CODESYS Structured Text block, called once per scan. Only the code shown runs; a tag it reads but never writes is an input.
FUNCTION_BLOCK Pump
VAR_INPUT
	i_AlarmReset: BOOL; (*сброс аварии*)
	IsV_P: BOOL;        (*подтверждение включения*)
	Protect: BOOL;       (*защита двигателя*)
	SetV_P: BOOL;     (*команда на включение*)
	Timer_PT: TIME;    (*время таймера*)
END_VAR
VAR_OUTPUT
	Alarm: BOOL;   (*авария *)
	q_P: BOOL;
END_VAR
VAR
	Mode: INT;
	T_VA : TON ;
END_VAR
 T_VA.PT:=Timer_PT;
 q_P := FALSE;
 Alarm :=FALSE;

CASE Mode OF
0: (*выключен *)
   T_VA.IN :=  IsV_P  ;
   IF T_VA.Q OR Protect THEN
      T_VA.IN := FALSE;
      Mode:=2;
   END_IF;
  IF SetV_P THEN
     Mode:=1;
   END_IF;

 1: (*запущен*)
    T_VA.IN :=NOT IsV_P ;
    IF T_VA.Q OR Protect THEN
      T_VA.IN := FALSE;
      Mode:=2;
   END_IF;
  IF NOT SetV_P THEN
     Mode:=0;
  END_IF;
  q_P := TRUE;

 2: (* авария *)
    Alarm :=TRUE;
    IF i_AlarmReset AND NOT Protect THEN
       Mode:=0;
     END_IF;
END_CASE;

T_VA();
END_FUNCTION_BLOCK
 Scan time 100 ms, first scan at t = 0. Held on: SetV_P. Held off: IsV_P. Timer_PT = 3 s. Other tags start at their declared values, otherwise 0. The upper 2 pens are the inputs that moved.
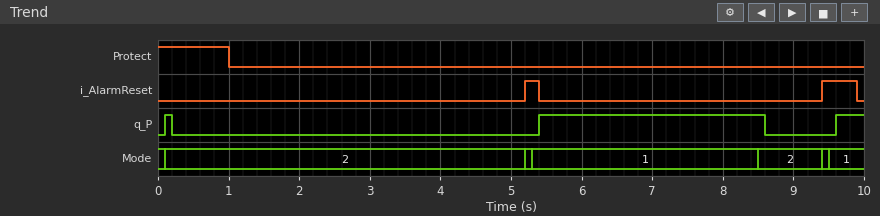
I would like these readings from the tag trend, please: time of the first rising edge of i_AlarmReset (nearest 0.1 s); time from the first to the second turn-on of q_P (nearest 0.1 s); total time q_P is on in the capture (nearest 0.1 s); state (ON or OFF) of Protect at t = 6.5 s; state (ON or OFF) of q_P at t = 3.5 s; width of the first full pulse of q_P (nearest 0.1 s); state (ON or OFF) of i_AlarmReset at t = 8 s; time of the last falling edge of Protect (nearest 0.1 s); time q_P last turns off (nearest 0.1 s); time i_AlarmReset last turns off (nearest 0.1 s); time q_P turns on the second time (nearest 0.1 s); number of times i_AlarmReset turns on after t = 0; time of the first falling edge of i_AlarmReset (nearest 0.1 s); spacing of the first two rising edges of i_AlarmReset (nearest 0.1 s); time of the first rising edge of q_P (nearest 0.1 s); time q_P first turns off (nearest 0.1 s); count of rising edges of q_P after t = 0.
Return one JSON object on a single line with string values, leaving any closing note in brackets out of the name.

{"time of the first rising edge of i_AlarmReset": "5.2 s", "time from the first to the second turn-on of q_P": "5.3 s", "total time q_P is on in the capture": "3.7 s", "state (ON or OFF) of Protect at t = 6.5 s": "OFF", "state (ON or OFF) of q_P at t = 3.5 s": "OFF", "width of the first full pulse of q_P": "0.1 s", "state (ON or OFF) of i_AlarmReset at t = 8 s": "OFF", "time of the last falling edge of Protect": "1.0 s", "time q_P last turns off": "8.6 s", "time i_AlarmReset last turns off": "9.9 s", "time q_P turns on the second time": "5.4 s", "number of times i_AlarmReset turns on after t = 0": "2", "time of the first falling edge of i_AlarmReset": "5.4 s", "spacing of the first two rising edges of i_AlarmReset": "4.2 s", "time of the first rising edge of q_P": "0.1 s", "time q_P first turns off": "0.2 s", "count of rising edges of q_P after t = 0": "3"}
